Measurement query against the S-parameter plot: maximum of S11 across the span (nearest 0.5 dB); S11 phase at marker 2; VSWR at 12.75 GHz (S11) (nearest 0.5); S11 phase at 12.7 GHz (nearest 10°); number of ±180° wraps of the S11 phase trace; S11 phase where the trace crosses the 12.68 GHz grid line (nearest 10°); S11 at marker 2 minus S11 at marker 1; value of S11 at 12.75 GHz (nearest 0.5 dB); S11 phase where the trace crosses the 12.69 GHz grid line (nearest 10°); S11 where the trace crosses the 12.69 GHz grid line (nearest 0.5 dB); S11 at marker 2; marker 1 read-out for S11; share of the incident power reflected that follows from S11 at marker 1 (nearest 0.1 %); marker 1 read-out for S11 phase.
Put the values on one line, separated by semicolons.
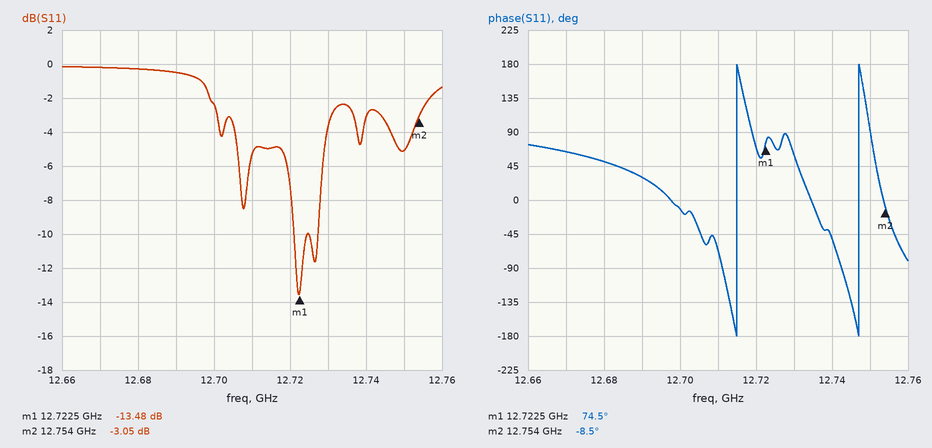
0.0 dB; -8.5°; 3.5; -10°; 2; 50°; 10.43 dB; -5.0 dB; 30°; -0.5 dB; -3.05 dB; -13.48 dB; 4.5 %; 74.5°
